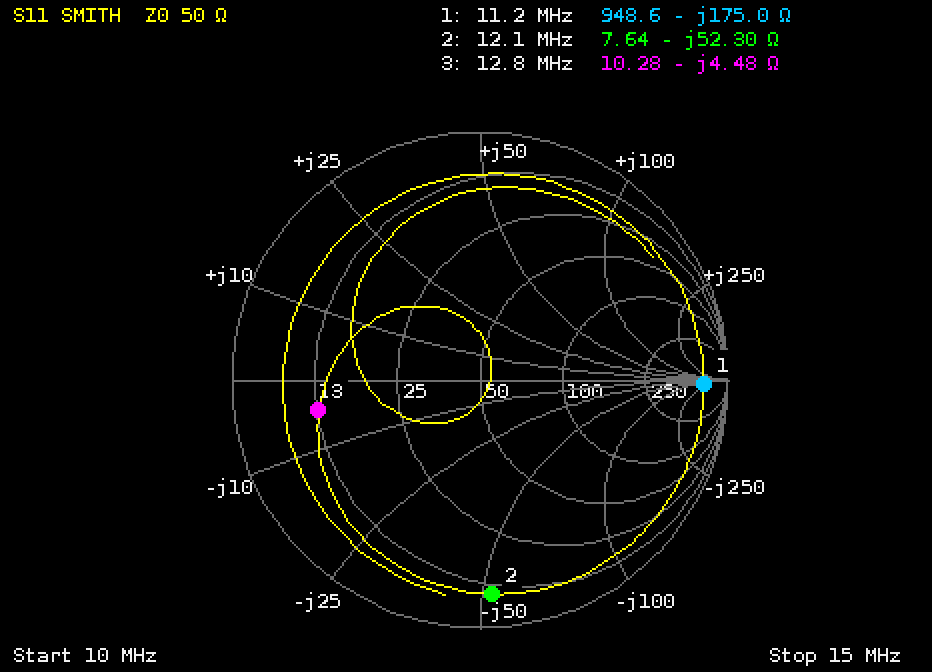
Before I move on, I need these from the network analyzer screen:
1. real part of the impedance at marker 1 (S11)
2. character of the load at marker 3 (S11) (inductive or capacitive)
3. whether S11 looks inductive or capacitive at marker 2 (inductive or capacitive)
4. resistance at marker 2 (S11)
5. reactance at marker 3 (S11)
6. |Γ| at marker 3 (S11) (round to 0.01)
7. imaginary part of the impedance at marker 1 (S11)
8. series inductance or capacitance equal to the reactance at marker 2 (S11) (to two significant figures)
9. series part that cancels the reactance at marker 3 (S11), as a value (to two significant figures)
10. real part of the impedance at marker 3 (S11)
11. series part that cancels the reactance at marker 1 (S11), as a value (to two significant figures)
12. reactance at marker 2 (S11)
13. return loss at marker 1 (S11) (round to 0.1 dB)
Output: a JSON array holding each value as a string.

["948.6 Ω", "capacitive", "capacitive", "7.64 Ω", "-4.48 Ω", "0.66", "-175.0 Ω", "250 pF", "56 nH", "10.28 Ω", "2.5 µH", "-52.30 Ω", "0.9 dB"]
